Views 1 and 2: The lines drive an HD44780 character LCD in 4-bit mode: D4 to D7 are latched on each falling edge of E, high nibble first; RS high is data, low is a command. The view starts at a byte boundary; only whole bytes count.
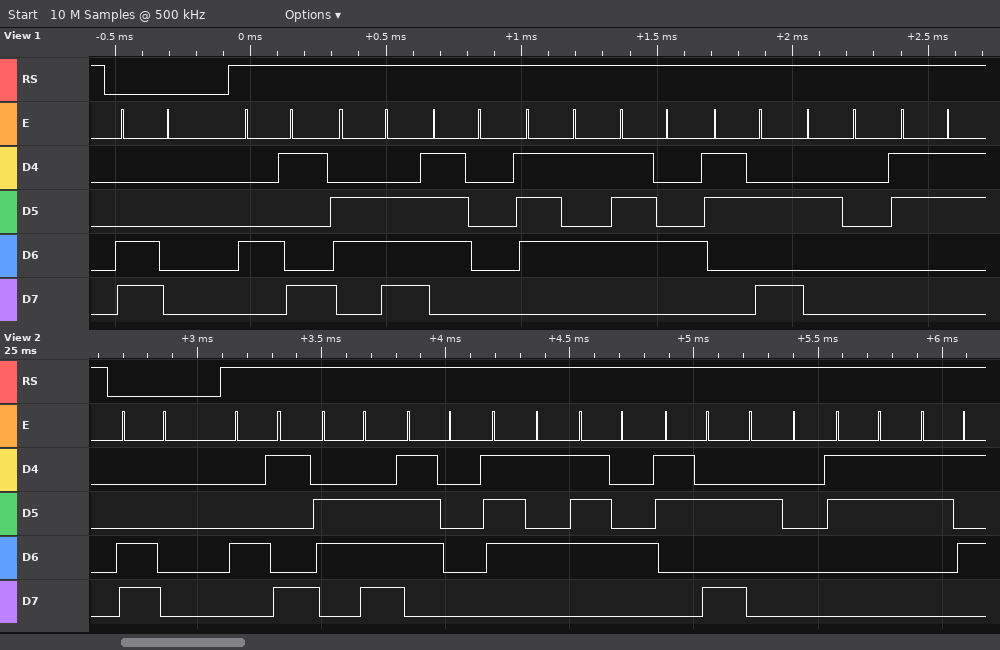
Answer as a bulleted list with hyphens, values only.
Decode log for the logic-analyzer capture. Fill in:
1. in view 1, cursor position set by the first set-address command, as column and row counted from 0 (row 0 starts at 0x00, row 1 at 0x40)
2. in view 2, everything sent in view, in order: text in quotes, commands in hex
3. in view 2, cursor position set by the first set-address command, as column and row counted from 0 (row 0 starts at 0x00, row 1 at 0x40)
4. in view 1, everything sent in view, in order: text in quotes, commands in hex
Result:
- column 0, row 1
- 0xC0 "Input: 35"
- column 0, row 1
- 0xC0 "Input: 3"
